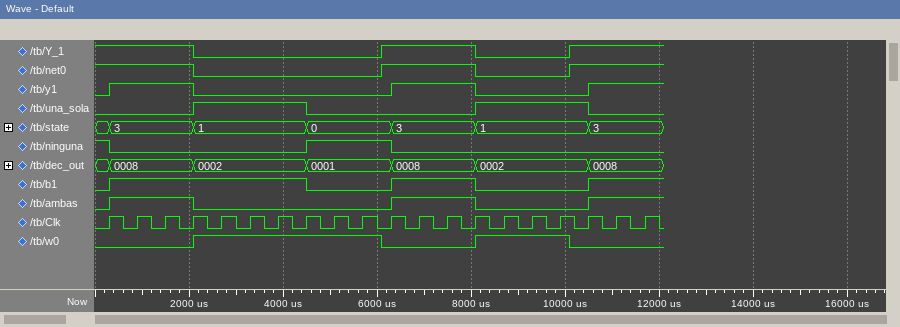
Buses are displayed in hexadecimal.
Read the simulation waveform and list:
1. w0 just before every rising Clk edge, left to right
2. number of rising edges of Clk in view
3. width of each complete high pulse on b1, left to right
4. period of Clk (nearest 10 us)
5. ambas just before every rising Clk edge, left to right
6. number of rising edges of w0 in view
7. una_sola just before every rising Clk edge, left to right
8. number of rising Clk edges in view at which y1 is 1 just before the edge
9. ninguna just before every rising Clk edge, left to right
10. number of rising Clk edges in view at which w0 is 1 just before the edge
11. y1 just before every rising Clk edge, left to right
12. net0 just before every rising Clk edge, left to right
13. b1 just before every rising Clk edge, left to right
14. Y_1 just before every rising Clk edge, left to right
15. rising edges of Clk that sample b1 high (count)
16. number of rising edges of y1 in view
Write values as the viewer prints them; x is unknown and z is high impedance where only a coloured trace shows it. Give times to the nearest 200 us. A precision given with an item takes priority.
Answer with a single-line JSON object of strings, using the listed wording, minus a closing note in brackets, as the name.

{"w0 just before every rising Clk edge, left to right": "0 0 0 0 1 1 1 1 1 1 0 0 0 0 1 1 1 0 0 0", "number of rising edges of Clk in view": "20", "width of each complete high pulse on b1, left to right": "4200 us, 1800 us", "period of Clk": "600 us", "ambas just before every rising Clk edge, left to right": "0 1 1 1 0 0 0 0 0 0 0 1 1 1 0 0 0 0 1 1", "number of rising edges of w0 in view": "2", "una_sola just before every rising Clk edge, left to right": "0 0 0 0 1 1 1 1 0 0 0 0 0 0 1 1 1 1 0 0", "number of rising Clk edges in view at which y1 is 1 just before the edge": "8", "ninguna just before every rising Clk edge, left to right": "1 0 0 0 0 0 0 0 1 1 1 0 0 0 0 0 0 0 0 0", "number of rising Clk edges in view at which w0 is 1 just before the edge": "9", "y1 just before every rising Clk edge, left to right": "0 1 1 1 0 0 0 0 0 0 0 1 1 1 0 0 0 0 1 1", "net0 just before every rising Clk edge, left to right": "1 1 1 1 0 0 0 0 0 0 1 1 1 1 0 0 0 1 1 1", "b1 just before every rising Clk edge, left to right": "0 1 1 1 1 1 1 1 0 0 0 1 1 1 0 0 0 0 1 1", "Y_1 just before every rising Clk edge, left to right": "1 1 1 1 0 0 0 0 0 0 1 1 1 1 0 0 0 1 1 1", "rising edges of Clk that sample b1 high": "12", "number of rising edges of y1 in view": "3"}
